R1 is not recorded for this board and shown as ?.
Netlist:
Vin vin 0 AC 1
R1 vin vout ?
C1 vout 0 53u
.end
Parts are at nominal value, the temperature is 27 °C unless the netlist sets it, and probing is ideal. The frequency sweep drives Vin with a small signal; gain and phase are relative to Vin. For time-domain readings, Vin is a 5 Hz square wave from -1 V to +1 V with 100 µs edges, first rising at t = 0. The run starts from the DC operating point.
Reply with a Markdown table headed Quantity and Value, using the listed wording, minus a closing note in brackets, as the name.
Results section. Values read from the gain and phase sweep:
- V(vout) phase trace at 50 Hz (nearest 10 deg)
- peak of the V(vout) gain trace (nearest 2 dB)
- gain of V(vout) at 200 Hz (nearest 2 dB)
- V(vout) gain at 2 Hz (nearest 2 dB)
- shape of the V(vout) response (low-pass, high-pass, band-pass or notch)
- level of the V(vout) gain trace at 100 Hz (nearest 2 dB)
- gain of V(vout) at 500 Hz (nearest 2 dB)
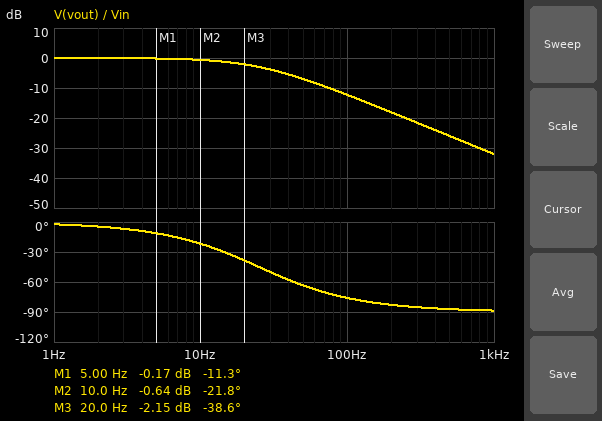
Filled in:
| Quantity | Value |
|---|---|
| V(vout) phase trace at 50 Hz | -60 deg |
| peak of the V(vout) gain trace | 0 dB |
| gain of V(vout) at 200 Hz | -18 dB |
| V(vout) gain at 2 Hz | 0 dB |
| shape of the V(vout) response | low-pass |
| level of the V(vout) gain trace at 100 Hz | -12 dB |
| gain of V(vout) at 500 Hz | -26 dB |
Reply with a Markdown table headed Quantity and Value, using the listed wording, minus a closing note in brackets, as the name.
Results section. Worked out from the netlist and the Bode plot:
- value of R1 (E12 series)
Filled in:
| Quantity | Value |
|---|---|
| value of R1 | 120 Ω |
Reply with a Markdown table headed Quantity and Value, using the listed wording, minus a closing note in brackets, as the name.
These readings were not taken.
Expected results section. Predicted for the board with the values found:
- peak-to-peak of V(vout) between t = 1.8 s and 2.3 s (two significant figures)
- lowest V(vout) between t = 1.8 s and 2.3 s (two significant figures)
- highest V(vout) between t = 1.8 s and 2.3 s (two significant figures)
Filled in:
| Quantity | Value |
|---|---|
| peak-to-peak of V(vout) between t = 1.8 s and 2.3 s | 2.0 V |
| lowest V(vout) between t = 1.8 s and 2.3 s | -1.0 V |
| highest V(vout) between t = 1.8 s and 2.3 s | 1.0 V |
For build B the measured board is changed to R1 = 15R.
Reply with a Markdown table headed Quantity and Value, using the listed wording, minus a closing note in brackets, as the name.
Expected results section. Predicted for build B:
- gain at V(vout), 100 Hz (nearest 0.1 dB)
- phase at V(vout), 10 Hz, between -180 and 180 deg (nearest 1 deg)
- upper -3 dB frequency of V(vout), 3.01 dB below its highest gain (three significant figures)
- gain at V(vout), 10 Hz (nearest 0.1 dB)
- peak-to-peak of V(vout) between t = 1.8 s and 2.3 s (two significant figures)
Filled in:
| Quantity | Value |
|---|---|
| gain at V(vout), 100 Hz | -1.0 dB |
| phase at V(vout), 10 Hz, between -180 and 180 deg | -3 deg |
| upper -3 dB frequency of V(vout), 3.01 dB below its highest gain | 200 Hz |
| gain at V(vout), 10 Hz | 0 dB |
| peak-to-peak of V(vout) between t = 1.8 s and 2.3 s | 2.0 V |
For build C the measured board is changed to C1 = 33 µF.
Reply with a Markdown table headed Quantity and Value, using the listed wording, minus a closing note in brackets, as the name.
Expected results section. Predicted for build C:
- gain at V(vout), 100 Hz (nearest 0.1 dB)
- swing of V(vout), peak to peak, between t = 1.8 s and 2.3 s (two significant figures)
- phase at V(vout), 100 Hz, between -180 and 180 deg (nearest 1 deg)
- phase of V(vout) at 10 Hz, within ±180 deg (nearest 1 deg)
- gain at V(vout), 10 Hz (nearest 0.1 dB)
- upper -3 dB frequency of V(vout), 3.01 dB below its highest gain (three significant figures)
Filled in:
| Quantity | Value |
|---|---|
| gain at V(vout), 100 Hz | -8.6 dB |
| swing of V(vout), peak to peak, between t = 1.8 s and 2.3 s | 2.0 V |
| phase at V(vout), 100 Hz, between -180 and 180 deg | -68 deg |
| phase of V(vout) at 10 Hz, within ±180 deg | -14 deg |
| gain at V(vout), 10 Hz | -0.3 dB |
| upper -3 dB frequency of V(vout), 3.01 dB below its highest gain | 40.2 Hz |
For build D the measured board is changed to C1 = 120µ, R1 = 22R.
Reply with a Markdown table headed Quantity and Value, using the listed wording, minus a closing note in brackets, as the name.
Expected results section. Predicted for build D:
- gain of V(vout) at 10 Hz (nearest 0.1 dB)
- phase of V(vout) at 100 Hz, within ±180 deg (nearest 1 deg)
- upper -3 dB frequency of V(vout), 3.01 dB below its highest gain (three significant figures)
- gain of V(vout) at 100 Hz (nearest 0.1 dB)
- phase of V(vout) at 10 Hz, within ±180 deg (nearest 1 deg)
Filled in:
| Quantity | Value |
|---|---|
| gain of V(vout) at 10 Hz | -0.1 dB |
| phase of V(vout) at 100 Hz, within ±180 deg | -59 deg |
| upper -3 dB frequency of V(vout), 3.01 dB below its highest gain | 60.3 Hz |
| gain of V(vout) at 100 Hz | -5.7 dB |
| phase of V(vout) at 10 Hz, within ±180 deg | -9 deg |
